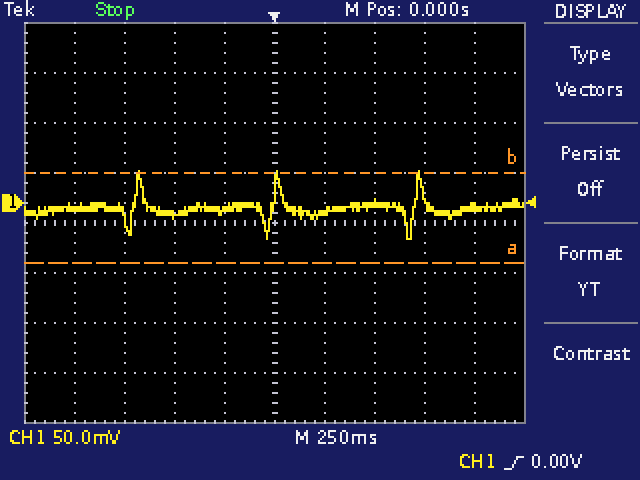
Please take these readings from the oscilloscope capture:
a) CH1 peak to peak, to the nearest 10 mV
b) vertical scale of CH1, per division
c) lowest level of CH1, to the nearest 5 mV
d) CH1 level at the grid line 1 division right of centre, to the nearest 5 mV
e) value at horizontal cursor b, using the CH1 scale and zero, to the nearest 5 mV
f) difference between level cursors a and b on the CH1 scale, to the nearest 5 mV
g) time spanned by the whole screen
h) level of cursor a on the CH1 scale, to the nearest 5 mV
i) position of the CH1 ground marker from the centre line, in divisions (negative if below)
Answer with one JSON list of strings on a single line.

["70 mV", "50 mV", "-35 mV", "-10 mV", "30 mV", "90 mV", "2.5 s", "-60 mV", "+0.4 div"]
